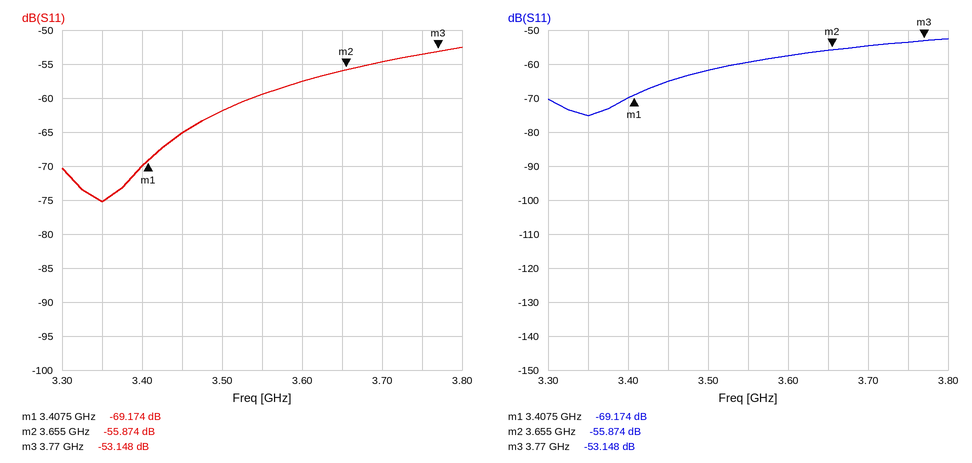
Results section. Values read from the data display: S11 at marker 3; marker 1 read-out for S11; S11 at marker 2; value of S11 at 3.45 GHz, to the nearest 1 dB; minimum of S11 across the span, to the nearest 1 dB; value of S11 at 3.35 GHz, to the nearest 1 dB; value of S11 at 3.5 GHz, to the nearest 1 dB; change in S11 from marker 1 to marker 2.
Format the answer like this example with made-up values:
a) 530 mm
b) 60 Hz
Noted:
a) -53.148 dB
b) -69.174 dB
c) -55.874 dB
d) -65 dB
e) -75 dB
f) -75 dB
g) -62 dB
h) 13.300 dB
